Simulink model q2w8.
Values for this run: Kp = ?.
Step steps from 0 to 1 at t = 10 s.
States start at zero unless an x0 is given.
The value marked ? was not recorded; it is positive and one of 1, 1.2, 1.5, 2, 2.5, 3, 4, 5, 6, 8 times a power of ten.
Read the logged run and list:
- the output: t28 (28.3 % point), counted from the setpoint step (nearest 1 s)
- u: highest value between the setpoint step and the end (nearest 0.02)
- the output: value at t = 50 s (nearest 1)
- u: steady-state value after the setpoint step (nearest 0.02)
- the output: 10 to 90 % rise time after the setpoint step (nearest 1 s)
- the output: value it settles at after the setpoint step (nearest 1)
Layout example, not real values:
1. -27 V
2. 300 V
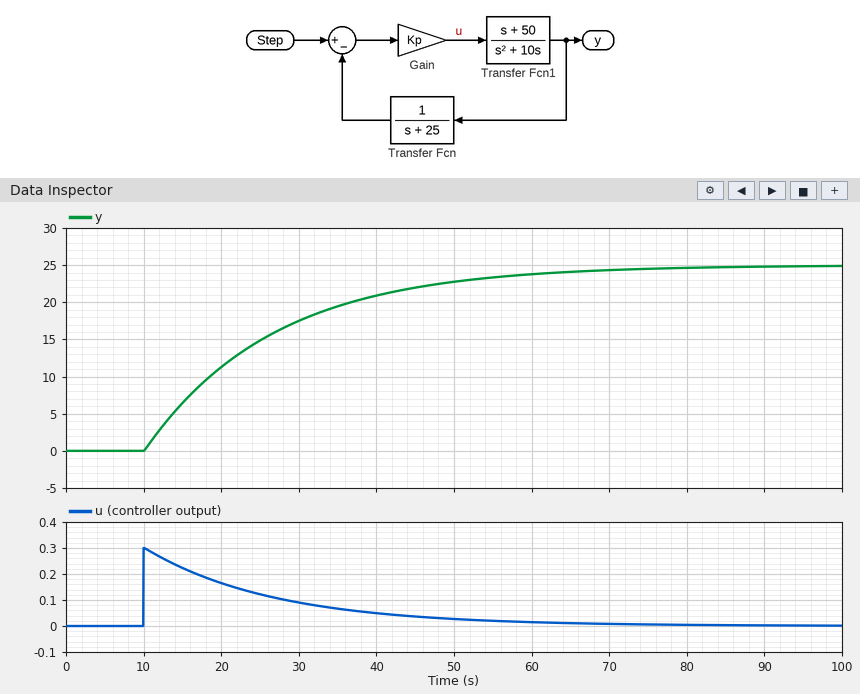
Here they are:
1. 6 s
2. 0.30
3. 23
4. 0.00
5. 36 s
6. 25
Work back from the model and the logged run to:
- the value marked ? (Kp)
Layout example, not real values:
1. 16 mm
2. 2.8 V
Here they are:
1. 0.3
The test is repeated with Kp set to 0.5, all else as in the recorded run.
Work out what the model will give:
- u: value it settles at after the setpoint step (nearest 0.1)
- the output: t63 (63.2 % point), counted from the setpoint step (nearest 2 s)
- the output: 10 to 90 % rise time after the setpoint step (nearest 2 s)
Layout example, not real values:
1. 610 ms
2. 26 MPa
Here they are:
1. 0.0
2. 10 s
3. 22 s
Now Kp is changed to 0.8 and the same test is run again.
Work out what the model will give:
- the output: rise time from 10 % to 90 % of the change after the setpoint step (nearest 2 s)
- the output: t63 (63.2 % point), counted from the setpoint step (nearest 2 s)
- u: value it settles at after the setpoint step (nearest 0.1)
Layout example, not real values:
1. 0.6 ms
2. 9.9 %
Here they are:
1. 14 s
2. 6 s
3. 0.0
